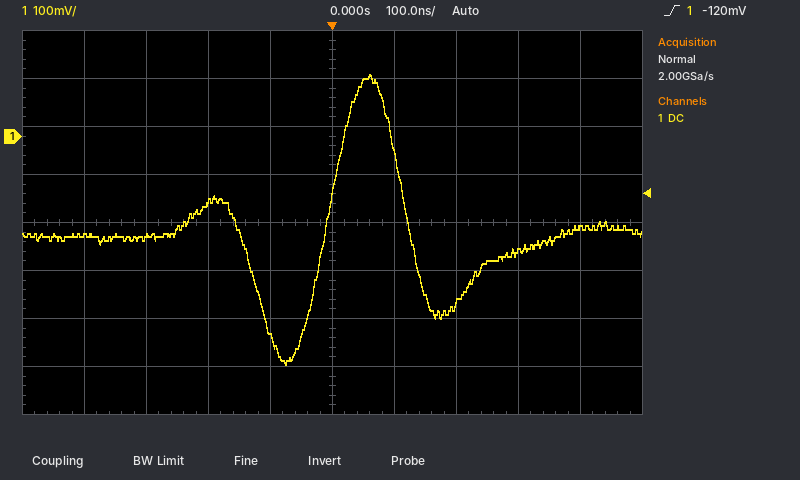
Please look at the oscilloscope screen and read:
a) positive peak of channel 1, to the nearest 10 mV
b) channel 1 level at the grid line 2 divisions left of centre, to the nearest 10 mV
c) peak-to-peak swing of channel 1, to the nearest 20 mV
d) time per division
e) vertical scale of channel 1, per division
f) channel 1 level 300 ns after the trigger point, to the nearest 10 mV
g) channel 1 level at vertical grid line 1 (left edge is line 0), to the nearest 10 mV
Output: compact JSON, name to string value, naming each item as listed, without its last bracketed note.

{"positive peak of channel 1, to the nearest 10 mV": "130 mV", "channel 1 level at the grid line 2 divisions left of centre, to the nearest 10 mV": "-140 mV", "peak-to-peak swing of channel 1, to the nearest 20 mV": "600 mV", "time per division": "100 ns", "vertical scale of channel 1, per division": "100 mV", "channel 1 level 300 ns after the trigger point, to the nearest 10 mV": "-240 mV", "channel 1 level at vertical grid line 1 (left edge is line 0), to the nearest 10 mV": "-210 mV"}
